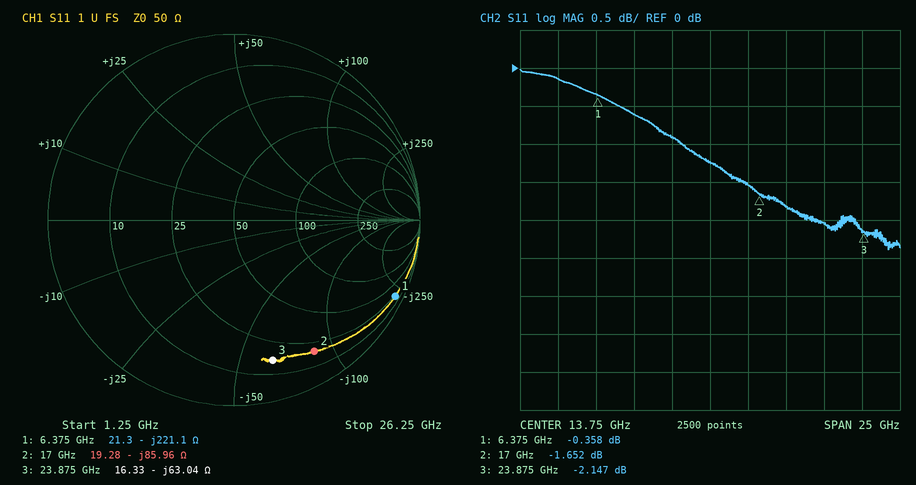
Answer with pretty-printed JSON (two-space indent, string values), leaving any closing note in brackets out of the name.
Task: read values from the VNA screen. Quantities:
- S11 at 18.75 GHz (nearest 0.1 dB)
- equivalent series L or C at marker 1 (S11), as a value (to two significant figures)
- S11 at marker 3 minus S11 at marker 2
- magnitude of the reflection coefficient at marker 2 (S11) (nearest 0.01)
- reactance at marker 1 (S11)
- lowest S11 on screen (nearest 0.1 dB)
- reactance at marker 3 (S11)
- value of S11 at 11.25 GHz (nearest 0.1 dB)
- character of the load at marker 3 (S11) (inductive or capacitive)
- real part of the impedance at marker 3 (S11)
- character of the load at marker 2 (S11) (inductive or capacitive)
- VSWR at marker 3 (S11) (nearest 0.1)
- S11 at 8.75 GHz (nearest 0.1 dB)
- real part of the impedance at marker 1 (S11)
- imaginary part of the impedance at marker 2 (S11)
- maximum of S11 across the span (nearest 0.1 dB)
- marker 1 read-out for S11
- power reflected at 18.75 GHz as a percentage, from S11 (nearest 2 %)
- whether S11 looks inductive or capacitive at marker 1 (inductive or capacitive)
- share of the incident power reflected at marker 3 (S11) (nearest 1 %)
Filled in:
{
  "S11 at 18.75 GHz": "-1.8 dB",
  "equivalent series L or C at marker 1 (S11), as a value": "110 fF",
  "S11 at marker 3 minus S11 at marker 2": "-0.495 dB",
  "magnitude of the reflection coefficient at marker 2 (S11)": "0.83",
  "reactance at marker 1": "-221.1 Ω",
  "lowest S11 on screen": "-2.4 dB",
  "reactance at marker 3": "-63.04 Ω",
  "value of S11 at 11.25 GHz": "-0.9 dB",
  "character of the load at marker 3 (S11)": "capacitive",
  "real part of the impedance at marker 3": "16.33 Ω",
  "character of the load at marker 2 (S11)": "capacitive",
  "VSWR at marker 3 (S11)": "8.1",
  "S11 at 8.75 GHz": "-0.6 dB",
  "real part of the impedance at marker 1": "21.3 Ω",
  "imaginary part of the impedance at marker 2": "-85.96 Ω",
  "maximum of S11 across the span": "0.0 dB",
  "marker 1 read-out for S11": "-0.358 dB",
  "power reflected at 18.75 GHz as a percentage, from S11": "66 %",
  "whether S11 looks inductive or capacitive at marker 1": "capacitive",
  "share of the incident power reflected at marker 3 (S11)": "61 %"
}
